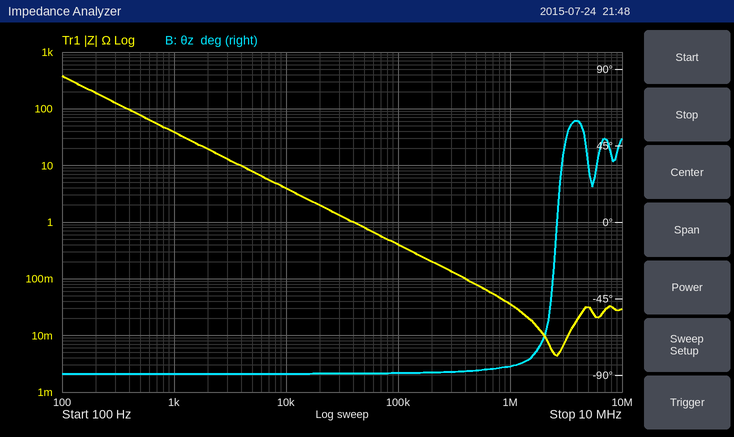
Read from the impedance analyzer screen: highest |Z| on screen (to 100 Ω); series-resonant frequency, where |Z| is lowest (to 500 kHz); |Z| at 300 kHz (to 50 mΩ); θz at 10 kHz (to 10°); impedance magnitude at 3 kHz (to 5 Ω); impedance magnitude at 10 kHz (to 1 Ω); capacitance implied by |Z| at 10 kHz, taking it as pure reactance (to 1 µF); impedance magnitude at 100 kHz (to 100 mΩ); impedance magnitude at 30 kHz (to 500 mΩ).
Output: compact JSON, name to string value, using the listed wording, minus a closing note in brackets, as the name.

{"highest |Z| on screen": "400 Ω", "series-resonant frequency, where |Z| is lowest": "2.5 MHz", "|Z| at 300 kHz": "150 mΩ", "θz at 10 kHz": "-90°", "impedance magnitude at 3 kHz": "15 Ω", "impedance magnitude at 10 kHz": "4 Ω", "capacitance implied by |Z| at 10 kHz, taking it as pure reactance": "4 µF", "impedance magnitude at 100 kHz": "400 mΩ", "impedance magnitude at 30 kHz": "1.5 Ω"}
